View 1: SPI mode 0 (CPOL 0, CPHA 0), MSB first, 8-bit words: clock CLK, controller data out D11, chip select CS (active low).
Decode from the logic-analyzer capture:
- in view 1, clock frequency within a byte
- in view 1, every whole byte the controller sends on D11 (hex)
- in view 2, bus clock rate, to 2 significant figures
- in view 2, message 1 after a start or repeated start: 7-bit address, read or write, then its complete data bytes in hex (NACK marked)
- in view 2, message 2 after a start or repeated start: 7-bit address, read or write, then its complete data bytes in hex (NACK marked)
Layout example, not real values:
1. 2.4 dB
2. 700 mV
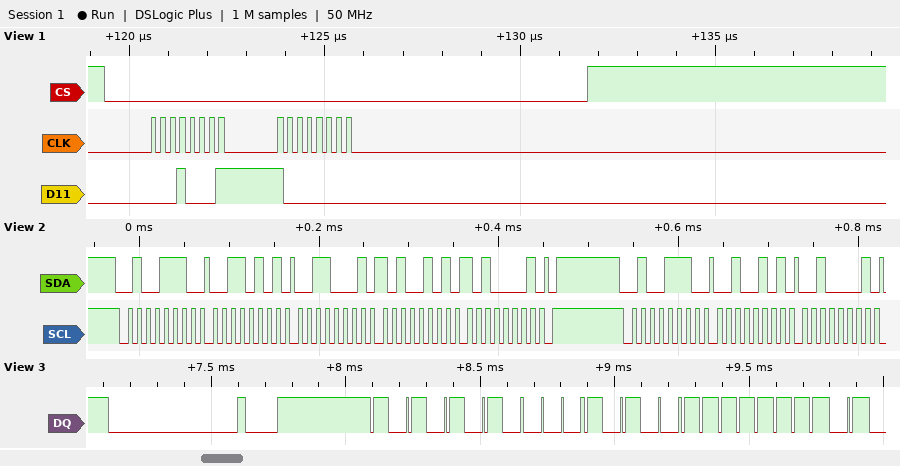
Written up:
1. 4 MHz
2. 11 80
3. 100 kHz
4. 0x27 write: 35 31 A5 A1
5. 0x27 write: 25 21
